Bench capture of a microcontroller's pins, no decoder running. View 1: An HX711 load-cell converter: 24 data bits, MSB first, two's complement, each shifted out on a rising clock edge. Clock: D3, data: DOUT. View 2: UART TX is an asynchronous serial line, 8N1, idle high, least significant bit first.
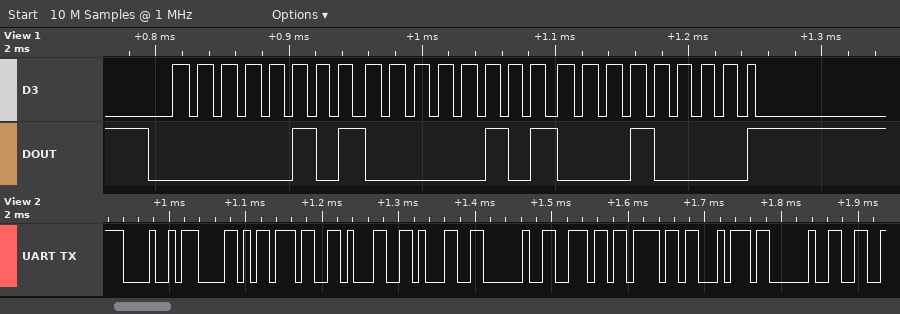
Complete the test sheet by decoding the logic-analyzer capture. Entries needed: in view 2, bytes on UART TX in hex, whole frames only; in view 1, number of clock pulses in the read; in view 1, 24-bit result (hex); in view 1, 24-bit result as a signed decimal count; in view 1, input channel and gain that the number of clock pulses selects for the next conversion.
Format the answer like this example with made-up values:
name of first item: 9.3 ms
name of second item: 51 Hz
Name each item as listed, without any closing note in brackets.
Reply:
in view 2, bytes on UART TX in hex, whole frames only: 48 58 37 31 31 20 6E 6F 74 20
in view 1, number of clock pulses in the read: 25
in view 1, 24-bit result: 0x050510
in view 1, 24-bit result as a signed decimal count: 328976
in view 1, input channel and gain that the number of clock pulses selects for the next conversion: channel A, gain 128
